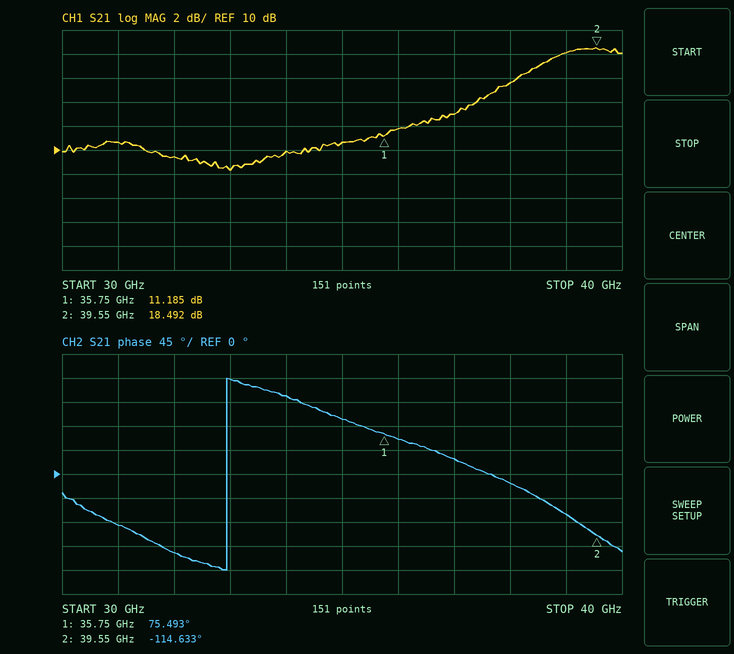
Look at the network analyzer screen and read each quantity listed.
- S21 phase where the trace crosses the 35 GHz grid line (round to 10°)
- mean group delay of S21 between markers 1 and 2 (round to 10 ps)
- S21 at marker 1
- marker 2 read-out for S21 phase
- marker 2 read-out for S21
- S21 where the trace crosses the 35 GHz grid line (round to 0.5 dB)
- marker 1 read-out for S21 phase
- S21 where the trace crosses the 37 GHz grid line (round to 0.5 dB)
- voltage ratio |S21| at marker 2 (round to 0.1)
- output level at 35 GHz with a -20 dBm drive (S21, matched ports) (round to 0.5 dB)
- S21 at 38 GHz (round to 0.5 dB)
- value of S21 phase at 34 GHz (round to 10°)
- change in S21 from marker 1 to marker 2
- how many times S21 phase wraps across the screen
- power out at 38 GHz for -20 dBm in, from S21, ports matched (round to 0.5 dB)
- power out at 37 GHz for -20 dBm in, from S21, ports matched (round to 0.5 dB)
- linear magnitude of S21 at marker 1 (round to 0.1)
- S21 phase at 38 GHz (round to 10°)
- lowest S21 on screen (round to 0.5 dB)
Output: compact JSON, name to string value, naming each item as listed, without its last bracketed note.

{"S21 phase where the trace crosses the 35 GHz grid line": "100°", "mean group delay of S21 between markers 1 and 2": "140 ps", "S21 at marker 1": "11.185 dB", "marker 2 read-out for S21 phase": "-114.633°", "marker 2 read-out for S21": "18.492 dB", "S21 where the trace crosses the 35 GHz grid line": "10.5 dB", "marker 1 read-out for S21 phase": "75.493°", "S21 where the trace crosses the 37 GHz grid line": "13.0 dB", "voltage ratio |S21| at marker 2": "8.4", "output level at 35 GHz with a -20 dBm drive (S21, matched ports)": "-9.5 dBm", "S21 at 38 GHz": "15.5 dB", "value of S21 phase at 34 GHz": "150°", "change in S21 from marker 1 to marker 2": "7.307 dB", "how many times S21 phase wraps across the screen": "1", "power out at 38 GHz for -20 dBm in, from S21, ports matched": "-4.5 dBm", "power out at 37 GHz for -20 dBm in, from S21, ports matched": "-7.0 dBm", "linear magnitude of S21 at marker 1": "3.6", "S21 phase at 38 GHz": "-20°", "lowest S21 on screen": "8.5 dB"}
